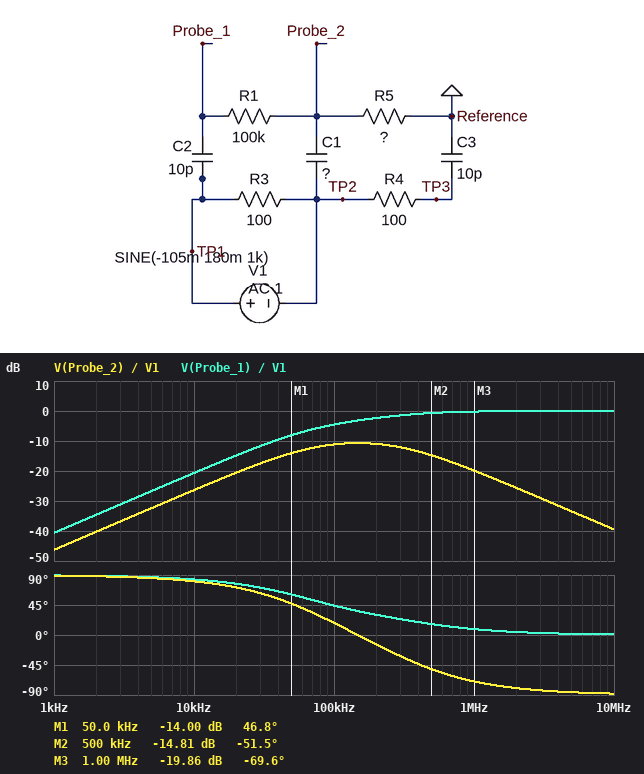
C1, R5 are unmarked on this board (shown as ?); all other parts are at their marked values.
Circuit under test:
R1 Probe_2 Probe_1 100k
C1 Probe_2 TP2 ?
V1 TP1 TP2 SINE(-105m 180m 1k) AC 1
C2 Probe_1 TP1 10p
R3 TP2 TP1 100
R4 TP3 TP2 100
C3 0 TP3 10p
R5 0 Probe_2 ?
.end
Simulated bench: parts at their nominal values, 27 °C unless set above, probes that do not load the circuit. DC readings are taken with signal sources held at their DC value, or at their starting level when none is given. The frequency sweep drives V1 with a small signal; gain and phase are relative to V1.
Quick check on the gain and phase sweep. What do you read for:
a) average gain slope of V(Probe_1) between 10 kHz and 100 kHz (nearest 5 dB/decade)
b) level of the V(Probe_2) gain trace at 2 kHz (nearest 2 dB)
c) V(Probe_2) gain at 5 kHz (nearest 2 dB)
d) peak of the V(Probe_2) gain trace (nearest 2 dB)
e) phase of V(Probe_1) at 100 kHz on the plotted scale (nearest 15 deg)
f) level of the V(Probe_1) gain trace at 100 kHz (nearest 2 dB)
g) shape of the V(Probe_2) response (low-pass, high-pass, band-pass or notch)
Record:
15 dB/decade
-40 dB
-32 dB
-10 dB
45 deg
-4 dB
band-pass
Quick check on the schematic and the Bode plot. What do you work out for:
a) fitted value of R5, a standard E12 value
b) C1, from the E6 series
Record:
270 kΩ
15 pF
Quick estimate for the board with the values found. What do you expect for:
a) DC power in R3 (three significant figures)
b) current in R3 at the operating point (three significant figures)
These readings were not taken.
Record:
110 µW
1.05 mA
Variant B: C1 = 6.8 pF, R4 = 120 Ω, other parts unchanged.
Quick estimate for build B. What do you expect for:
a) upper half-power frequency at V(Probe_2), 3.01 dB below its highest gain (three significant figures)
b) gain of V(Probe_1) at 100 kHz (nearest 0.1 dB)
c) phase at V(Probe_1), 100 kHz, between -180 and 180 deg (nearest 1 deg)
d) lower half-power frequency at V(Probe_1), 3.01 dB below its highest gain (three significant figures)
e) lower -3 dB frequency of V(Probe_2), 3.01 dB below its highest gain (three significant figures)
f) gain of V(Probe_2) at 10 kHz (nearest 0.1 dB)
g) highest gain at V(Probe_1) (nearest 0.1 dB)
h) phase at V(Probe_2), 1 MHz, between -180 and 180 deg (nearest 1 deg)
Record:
600 kHz
-3.7 dB
41 deg
125 kHz
61.6 kHz
-24.0 dB
0 dB
-61 deg
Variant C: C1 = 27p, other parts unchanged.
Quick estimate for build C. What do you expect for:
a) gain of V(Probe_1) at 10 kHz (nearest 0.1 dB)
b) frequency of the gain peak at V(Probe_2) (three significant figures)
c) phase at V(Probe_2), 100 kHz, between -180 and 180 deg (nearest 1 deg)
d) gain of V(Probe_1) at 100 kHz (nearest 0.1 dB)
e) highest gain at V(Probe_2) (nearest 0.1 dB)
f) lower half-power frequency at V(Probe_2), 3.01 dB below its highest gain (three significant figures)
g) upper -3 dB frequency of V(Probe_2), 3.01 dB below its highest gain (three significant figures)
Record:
-21.4 dB
128 kHz
12 deg
-5.0 dB
-14.1 dB
47.2 kHz
346 kHz
